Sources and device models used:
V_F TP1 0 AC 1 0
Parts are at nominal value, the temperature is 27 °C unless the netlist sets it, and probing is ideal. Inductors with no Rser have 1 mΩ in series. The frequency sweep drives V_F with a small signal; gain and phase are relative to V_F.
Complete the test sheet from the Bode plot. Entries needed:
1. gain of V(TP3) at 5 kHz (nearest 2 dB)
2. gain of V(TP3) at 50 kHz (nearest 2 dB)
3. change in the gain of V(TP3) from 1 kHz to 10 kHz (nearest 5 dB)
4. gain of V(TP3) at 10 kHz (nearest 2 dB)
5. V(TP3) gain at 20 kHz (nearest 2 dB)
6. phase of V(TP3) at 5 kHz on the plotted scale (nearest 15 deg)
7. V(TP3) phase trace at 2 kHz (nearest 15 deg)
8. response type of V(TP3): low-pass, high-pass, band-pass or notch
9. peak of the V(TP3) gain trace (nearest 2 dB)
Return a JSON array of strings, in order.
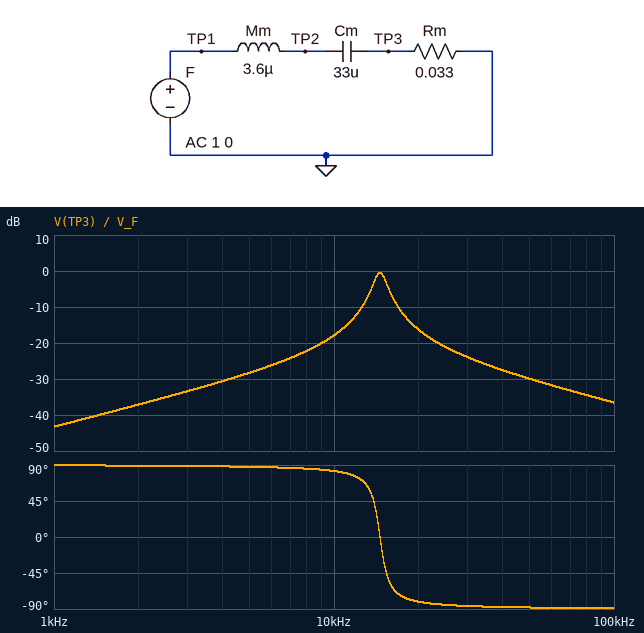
["-28 dB", "-30 dB", "25 dB", "-18 dB", "-16 dB", "90 deg", "90 deg", "band-pass", "0 dB"]
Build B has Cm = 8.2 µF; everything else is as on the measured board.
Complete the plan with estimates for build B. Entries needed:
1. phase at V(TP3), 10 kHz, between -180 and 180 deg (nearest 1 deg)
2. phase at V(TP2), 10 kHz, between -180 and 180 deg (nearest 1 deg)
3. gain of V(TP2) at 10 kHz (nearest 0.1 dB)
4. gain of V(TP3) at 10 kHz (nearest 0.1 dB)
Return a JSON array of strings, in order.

["89 deg", "0 deg", "1.1 dB", "-34.3 dB"]
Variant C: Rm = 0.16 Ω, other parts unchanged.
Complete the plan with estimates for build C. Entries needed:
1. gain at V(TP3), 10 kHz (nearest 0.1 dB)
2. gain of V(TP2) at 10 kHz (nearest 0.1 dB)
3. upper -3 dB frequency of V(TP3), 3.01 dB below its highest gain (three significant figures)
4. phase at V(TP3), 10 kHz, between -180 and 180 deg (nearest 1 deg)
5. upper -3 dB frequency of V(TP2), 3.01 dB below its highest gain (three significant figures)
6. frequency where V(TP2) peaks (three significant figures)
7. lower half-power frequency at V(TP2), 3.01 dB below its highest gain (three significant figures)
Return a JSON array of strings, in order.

["-5.5 dB", "4.5 dB", "18.6 kHz", "58 deg", "17.3 kHz", "13.9 kHz", "9.80 kHz"]
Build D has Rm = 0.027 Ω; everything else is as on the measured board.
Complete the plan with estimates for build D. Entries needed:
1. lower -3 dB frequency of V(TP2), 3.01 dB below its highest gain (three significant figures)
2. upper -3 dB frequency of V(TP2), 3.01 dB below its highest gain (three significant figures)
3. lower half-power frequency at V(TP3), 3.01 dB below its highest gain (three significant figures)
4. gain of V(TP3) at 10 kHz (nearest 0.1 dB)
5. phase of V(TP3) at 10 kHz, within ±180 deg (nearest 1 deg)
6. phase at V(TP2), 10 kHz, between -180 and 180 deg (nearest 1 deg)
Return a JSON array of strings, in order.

["13.9 kHz", "15.2 kHz", "14.0 kHz", "-19.6 dB", "84 deg", "-3 deg"]
